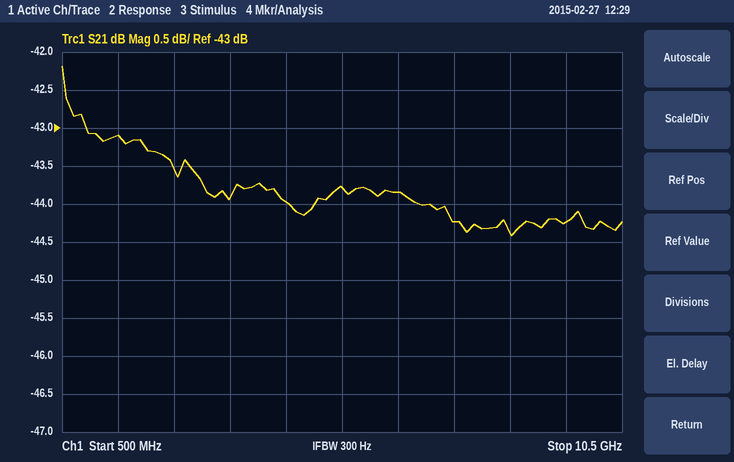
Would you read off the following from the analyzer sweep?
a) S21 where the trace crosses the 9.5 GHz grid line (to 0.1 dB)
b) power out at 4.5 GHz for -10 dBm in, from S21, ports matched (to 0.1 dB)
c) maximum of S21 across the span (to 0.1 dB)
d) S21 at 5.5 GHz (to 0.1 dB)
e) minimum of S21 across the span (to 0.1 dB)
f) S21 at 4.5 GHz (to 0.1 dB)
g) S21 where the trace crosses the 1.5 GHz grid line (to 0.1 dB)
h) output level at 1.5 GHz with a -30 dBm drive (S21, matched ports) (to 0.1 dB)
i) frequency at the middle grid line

-44.2 dB
-54.0 dBm
-42.2 dB
-43.8 dB
-44.4 dB
-44.0 dB
-43.1 dB
-73.1 dBm
5.5 GHz
